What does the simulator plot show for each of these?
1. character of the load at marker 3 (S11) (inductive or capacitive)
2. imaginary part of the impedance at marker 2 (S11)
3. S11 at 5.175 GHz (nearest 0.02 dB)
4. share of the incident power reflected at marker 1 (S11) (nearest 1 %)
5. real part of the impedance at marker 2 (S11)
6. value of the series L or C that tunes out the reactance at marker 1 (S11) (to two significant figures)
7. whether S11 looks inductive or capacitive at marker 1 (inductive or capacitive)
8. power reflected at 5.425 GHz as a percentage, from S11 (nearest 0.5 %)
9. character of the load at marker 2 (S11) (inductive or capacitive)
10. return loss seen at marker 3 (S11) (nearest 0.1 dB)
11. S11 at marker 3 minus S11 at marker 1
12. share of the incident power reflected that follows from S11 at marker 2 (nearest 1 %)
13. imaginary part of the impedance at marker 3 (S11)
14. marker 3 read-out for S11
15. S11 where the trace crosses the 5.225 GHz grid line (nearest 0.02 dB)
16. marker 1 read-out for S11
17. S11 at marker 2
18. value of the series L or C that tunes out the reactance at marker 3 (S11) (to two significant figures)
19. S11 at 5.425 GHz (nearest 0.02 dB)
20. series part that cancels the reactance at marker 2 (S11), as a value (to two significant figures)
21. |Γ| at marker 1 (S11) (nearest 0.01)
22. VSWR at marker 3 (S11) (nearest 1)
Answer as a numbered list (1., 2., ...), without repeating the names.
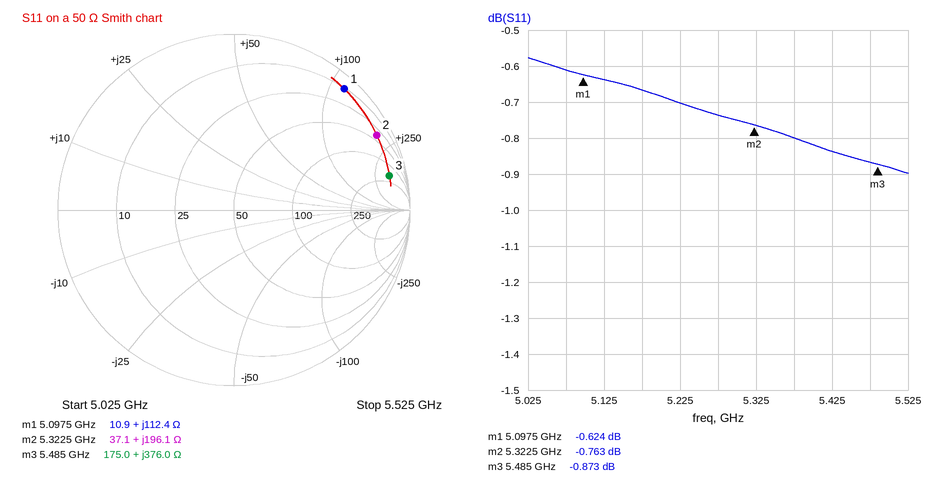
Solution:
1. inductive
2. +196.1 Ω
3. -0.66 dB
4. 87 %
5. 37.1 Ω
6. 280 fF
7. inductive
8. 82.5 %
9. inductive
10. 0.9 dB
11. -0.249 dB
12. 84 %
13. +376.0 Ω
14. -0.873 dB
15. -0.70 dB
16. -0.624 dB
17. -0.763 dB
18. 77 fF
19. -0.84 dB
20. 150 fF
21. 0.93
22. 20
